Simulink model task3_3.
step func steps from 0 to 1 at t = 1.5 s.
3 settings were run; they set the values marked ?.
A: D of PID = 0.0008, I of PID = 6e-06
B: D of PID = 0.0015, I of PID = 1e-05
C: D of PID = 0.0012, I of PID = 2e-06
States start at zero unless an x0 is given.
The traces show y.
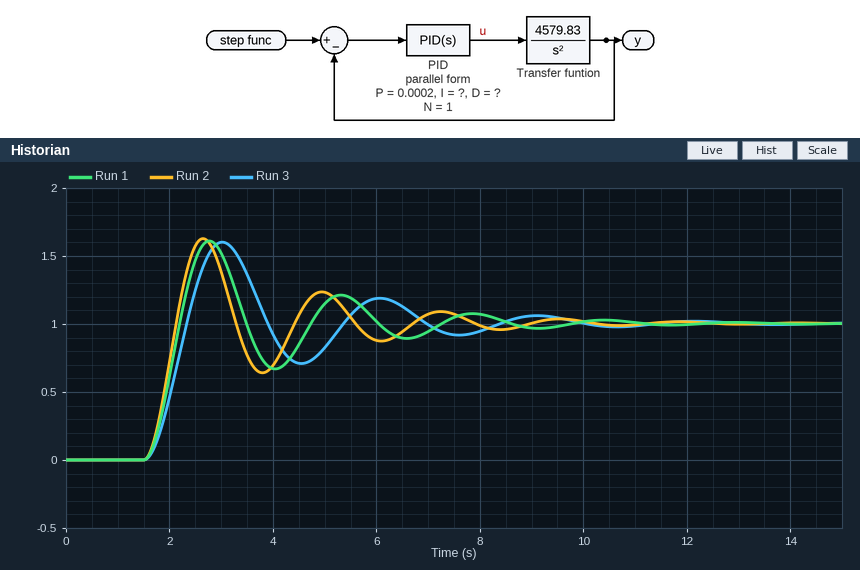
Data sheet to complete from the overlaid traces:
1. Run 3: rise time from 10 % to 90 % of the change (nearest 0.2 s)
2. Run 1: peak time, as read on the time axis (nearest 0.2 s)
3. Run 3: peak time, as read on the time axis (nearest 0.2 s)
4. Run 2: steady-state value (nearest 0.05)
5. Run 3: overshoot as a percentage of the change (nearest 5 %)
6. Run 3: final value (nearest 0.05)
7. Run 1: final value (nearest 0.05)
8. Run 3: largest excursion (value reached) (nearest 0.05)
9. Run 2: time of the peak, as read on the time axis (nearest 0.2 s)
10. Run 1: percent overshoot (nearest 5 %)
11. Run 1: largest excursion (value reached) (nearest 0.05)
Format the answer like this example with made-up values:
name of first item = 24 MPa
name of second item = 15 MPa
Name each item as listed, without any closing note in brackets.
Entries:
Run 3: rise time from 10 % to 90 % of the change = 0.6 s
Run 1: peak time, as read on the time axis = 2.8 s
Run 3: peak time, as read on the time axis = 3.0 s
Run 2: steady-state value = 1.00
Run 3: overshoot as a percentage of the change = 60 %
Run 3: final value = 1.00
Run 1: final value = 1.00
Run 3: largest excursion (value reached) = 1.60
Run 2: time of the peak, as read on the time axis = 2.6 s
Run 1: percent overshoot = 60 %
Run 1: largest excursion (value reached) = 1.60
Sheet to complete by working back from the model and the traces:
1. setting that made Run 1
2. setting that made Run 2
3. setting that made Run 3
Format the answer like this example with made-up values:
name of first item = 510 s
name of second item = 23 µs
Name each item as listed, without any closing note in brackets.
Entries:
setting that made Run 1 = C
setting that made Run 2 = B
setting that made Run 3 = A
